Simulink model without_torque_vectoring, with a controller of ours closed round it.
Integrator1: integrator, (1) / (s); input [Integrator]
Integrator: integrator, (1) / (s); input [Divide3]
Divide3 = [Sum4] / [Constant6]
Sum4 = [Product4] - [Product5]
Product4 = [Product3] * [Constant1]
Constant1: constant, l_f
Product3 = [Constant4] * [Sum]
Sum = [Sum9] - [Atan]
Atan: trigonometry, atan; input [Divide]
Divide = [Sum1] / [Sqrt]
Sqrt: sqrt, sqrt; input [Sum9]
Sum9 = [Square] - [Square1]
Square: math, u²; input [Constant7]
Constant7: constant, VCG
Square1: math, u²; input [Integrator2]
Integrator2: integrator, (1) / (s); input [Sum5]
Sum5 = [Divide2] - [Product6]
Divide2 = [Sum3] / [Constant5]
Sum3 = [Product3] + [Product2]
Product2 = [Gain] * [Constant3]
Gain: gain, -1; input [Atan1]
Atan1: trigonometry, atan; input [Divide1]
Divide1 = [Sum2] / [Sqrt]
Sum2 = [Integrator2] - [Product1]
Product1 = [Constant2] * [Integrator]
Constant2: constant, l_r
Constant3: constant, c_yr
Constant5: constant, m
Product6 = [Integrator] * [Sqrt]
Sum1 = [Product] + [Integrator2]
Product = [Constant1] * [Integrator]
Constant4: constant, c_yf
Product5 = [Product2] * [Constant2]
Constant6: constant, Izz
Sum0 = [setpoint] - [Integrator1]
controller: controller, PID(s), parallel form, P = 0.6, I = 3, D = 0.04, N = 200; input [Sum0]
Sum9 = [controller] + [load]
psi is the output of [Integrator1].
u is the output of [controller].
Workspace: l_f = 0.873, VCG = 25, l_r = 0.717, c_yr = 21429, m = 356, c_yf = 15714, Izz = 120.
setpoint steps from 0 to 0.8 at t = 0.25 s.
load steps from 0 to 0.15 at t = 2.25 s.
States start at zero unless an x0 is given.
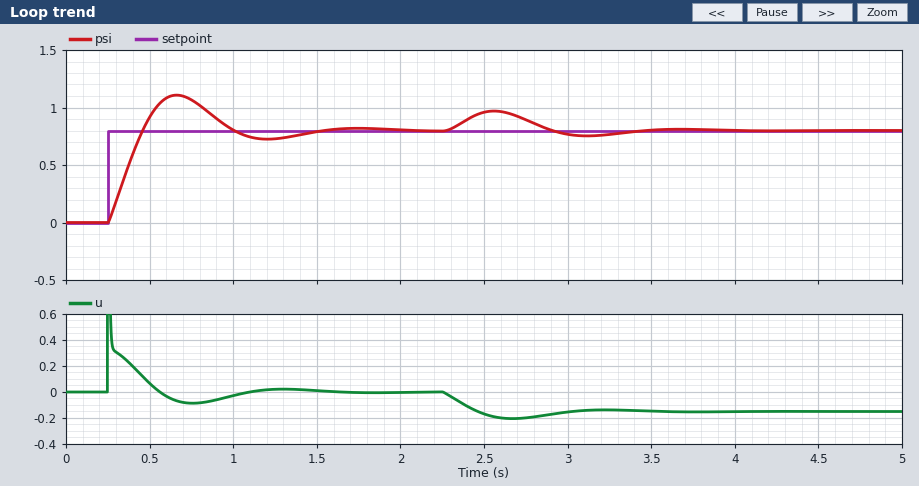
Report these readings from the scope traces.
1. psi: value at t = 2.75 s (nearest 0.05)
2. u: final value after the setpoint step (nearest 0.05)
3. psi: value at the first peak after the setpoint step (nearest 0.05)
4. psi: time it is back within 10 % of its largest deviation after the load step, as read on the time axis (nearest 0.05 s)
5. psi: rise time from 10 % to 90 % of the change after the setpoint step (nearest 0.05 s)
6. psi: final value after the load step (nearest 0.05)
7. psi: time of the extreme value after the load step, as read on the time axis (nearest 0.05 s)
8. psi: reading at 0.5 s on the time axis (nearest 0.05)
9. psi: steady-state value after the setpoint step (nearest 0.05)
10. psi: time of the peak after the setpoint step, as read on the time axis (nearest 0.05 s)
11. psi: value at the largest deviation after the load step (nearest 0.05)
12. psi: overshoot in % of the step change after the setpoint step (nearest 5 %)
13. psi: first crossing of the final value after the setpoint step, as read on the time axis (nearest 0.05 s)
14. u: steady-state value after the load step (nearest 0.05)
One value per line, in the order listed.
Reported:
0.90
0.00
1.10
3.35 s
0.15 s
0.80
2.55 s
0.90
0.80
0.65 s
0.95
40 %
0.45 s
-0.15
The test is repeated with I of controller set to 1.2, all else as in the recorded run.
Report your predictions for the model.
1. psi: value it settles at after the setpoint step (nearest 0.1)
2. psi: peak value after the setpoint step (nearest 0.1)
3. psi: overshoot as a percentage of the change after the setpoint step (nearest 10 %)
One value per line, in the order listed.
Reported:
0.8
0.9
20 %
